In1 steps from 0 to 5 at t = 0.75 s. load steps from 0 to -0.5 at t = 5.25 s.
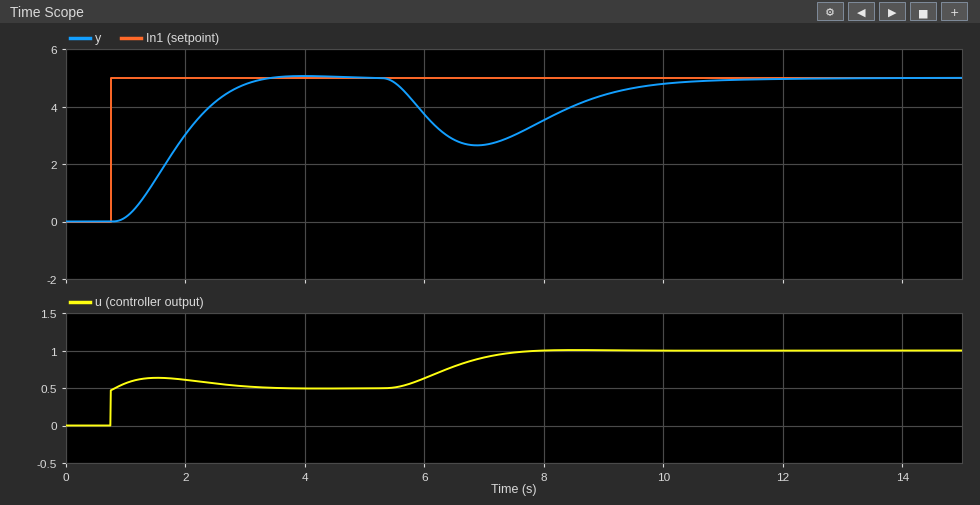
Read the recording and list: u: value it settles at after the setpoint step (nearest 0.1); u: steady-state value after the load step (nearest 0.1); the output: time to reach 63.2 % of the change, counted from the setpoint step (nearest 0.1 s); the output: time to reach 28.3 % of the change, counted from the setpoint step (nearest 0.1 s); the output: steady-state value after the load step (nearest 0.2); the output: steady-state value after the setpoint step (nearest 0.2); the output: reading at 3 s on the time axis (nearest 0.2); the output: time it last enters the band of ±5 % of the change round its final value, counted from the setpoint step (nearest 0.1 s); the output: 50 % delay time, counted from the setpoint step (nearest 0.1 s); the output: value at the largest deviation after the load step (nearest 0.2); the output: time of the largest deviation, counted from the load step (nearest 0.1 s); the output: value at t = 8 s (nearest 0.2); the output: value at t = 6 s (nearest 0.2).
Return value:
0.5
1.0
1.3 s
0.7 s
5.0
5.0
4.8
2.2 s
1.1 s
2.6
1.6 s
3.6
3.8
